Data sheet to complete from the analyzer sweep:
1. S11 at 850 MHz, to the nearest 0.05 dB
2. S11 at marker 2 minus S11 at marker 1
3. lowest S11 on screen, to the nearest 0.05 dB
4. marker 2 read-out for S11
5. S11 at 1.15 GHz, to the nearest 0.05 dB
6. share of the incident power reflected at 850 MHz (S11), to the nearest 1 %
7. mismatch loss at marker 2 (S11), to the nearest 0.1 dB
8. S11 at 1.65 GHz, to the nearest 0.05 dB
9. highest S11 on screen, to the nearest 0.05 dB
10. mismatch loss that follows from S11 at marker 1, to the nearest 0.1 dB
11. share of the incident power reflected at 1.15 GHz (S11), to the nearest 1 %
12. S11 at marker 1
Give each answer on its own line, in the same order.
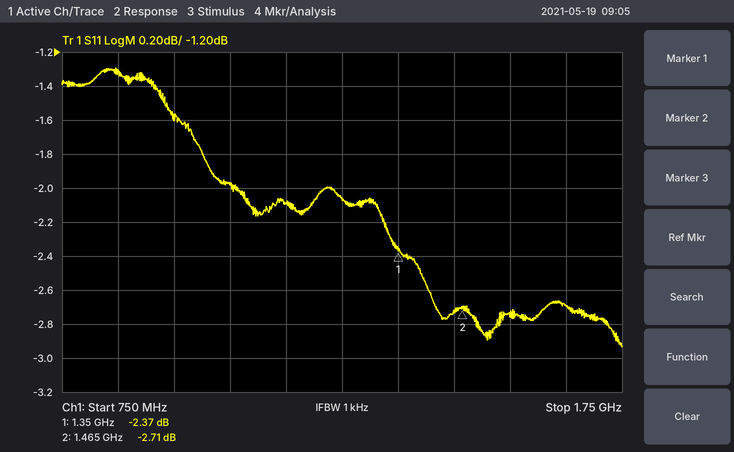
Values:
-1.30 dB
-0.34 dB
-2.95 dB
-2.71 dB
-2.10 dB
74 %
3.3 dB
-2.70 dB
-1.30 dB
3.8 dB
62 %
-2.37 dB
